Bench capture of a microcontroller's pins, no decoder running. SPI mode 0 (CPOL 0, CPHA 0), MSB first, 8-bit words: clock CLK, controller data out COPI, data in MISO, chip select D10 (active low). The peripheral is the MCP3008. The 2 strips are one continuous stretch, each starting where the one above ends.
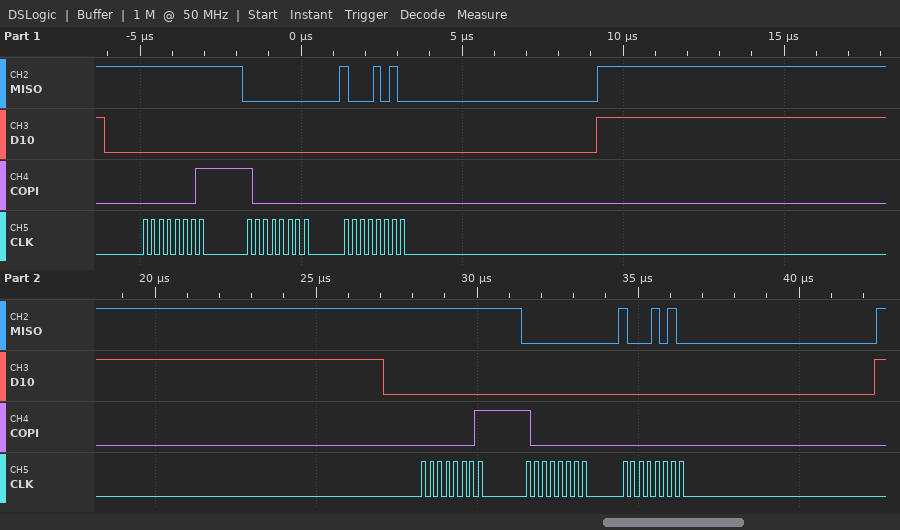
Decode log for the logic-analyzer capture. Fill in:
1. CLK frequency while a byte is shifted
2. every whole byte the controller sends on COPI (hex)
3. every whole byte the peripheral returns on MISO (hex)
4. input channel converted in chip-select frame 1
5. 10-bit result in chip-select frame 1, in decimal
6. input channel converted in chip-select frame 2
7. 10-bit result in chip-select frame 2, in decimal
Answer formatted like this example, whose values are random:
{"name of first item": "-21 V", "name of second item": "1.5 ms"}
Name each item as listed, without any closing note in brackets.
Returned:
{"CLK frequency while a byte is shifted": "4 MHz", "every whole byte the controller sends on COPI": "0x01 0x80 0x00 0x01 0x80 0x00", "every whole byte the peripheral returns on MISO": "0xFF 0x00 0x8A 0xFF 0x00 0x8A", "input channel converted in chip-select frame 1": "0", "10-bit result in chip-select frame 1, in decimal": "138", "input channel converted in chip-select frame 2": "0", "10-bit result in chip-select frame 2, in decimal": "138"}
